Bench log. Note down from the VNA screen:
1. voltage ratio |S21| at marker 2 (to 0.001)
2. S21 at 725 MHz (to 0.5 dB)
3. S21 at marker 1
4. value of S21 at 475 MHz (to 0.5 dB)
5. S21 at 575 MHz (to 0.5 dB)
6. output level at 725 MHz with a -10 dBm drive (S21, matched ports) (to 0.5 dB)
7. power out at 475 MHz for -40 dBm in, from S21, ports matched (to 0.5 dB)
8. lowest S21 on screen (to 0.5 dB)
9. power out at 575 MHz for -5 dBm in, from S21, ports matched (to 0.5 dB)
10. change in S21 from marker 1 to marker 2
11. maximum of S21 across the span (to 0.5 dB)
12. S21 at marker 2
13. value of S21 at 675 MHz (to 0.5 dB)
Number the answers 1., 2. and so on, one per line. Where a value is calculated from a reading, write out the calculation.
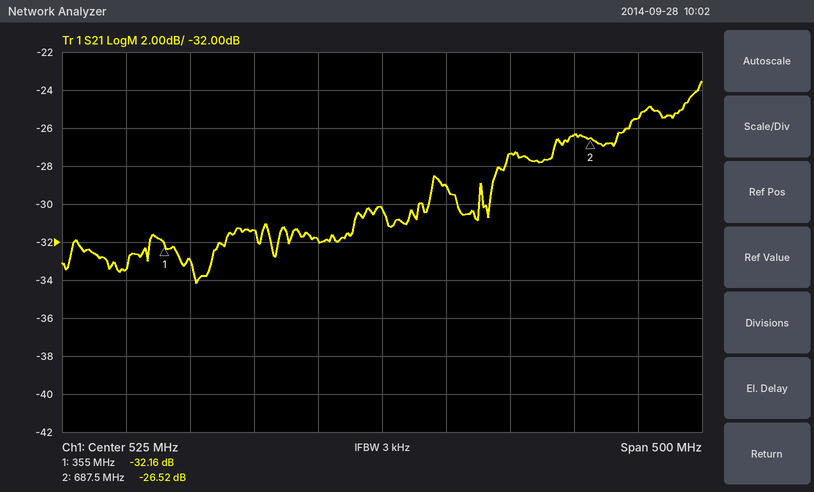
1. 10^(-26.52/20) ≈ 0.047
2. -25.5 dB
3. -32.16 dB
4. -32.0 dB
5. -29.0 dB
6. -10 dBm + (-25.5 dB) = -35.5 dBm
7. -40 dBm + (-32.0 dB) = -72.0 dBm
8. -34.0 dB
9. -5 dBm + (-29.0 dB) = -34.0 dBm
10. -26.52 − (-32.16) = 5.64 dB
11. -23.5 dB
12. -26.52 dB
13. -26.5 dB
